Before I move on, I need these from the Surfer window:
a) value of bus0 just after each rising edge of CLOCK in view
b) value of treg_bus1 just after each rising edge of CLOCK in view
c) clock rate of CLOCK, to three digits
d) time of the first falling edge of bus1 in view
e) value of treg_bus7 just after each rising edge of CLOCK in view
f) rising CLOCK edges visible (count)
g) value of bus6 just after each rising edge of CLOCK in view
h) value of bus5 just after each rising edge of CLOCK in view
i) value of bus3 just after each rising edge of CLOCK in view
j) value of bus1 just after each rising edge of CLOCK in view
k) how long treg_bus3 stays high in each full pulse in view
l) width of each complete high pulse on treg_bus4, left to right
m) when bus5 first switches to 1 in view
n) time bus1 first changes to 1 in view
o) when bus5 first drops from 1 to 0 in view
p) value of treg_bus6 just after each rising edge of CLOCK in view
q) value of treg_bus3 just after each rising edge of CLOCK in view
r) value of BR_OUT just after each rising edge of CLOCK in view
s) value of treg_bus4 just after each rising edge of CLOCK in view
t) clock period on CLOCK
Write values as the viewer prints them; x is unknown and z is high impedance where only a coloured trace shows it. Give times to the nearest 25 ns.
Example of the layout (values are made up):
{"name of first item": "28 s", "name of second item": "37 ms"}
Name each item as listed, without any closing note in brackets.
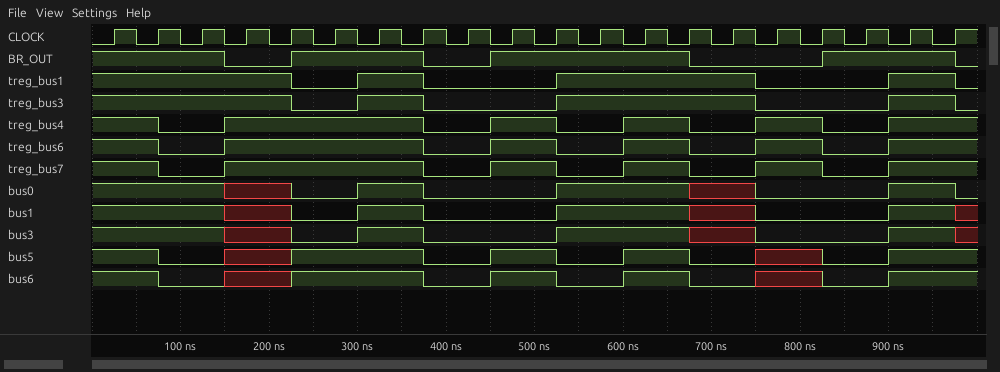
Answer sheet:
{"value of bus0 just after each rising edge of CLOCK in view": "1 1 1 x 0 0 1 0 0 0 1 1 1 x x 0 0 0 1 0", "value of treg_bus1 just after each rising edge of CLOCK in view": "1 1 1 1 0 0 1 0 0 0 1 1 1 1 1 0 0 0 1 0", "clock rate of CLOCK, to three digits": "20.0 MHz", "time of the first falling edge of bus1 in view": "375 ns", "value of treg_bus7 just after each rising edge of CLOCK in view": "1 0 0 1 1 1 1 0 0 1 0 0 1 0 0 1 0 0 1 1", "rising CLOCK edges visible": "20", "value of bus6 just after each rising edge of CLOCK in view": "1 0 0 x 1 1 1 0 0 1 0 0 1 0 0 x 0 0 1 1", "value of bus5 just after each rising edge of CLOCK in view": "1 0 0 x 1 1 1 0 0 1 0 0 1 0 0 x 0 0 1 1", "value of bus3 just after each rising edge of CLOCK in view": "1 1 1 x 0 0 1 0 0 0 1 1 1 x x 0 0 0 1 x", "value of bus1 just after each rising edge of CLOCK in view": "1 1 1 x 0 0 1 0 0 0 1 1 1 x x 0 0 0 1 x", "how long treg_bus3 stays high in each full pulse in view": "75 ns, 225 ns, 75 ns", "width of each complete high pulse on treg_bus4, left to right": "225 ns, 75 ns, 75 ns, 75 ns", "when bus5 first switches to 1 in view": "225 ns", "time bus1 first changes to 1 in view": "300 ns", "when bus5 first drops from 1 to 0 in view": "75 ns", "value of treg_bus6 just after each rising edge of CLOCK in view": "1 0 0 1 1 1 1 0 0 1 0 0 1 0 0 1 0 0 1 1", "value of treg_bus3 just after each rising edge of CLOCK in view": "1 1 1 1 0 0 1 0 0 0 1 1 1 1 1 0 0 0 1 0", "value of BR_OUT just after each rising edge of CLOCK in view": "1 1 1 0 1 1 1 0 0 1 1 1 1 0 0 0 1 1 1 0", "value of treg_bus4 just after each rising edge of CLOCK in view": "1 0 0 1 1 1 1 0 0 1 0 0 1 0 0 1 0 0 1 1", "clock period on CLOCK": "50 ns"}
